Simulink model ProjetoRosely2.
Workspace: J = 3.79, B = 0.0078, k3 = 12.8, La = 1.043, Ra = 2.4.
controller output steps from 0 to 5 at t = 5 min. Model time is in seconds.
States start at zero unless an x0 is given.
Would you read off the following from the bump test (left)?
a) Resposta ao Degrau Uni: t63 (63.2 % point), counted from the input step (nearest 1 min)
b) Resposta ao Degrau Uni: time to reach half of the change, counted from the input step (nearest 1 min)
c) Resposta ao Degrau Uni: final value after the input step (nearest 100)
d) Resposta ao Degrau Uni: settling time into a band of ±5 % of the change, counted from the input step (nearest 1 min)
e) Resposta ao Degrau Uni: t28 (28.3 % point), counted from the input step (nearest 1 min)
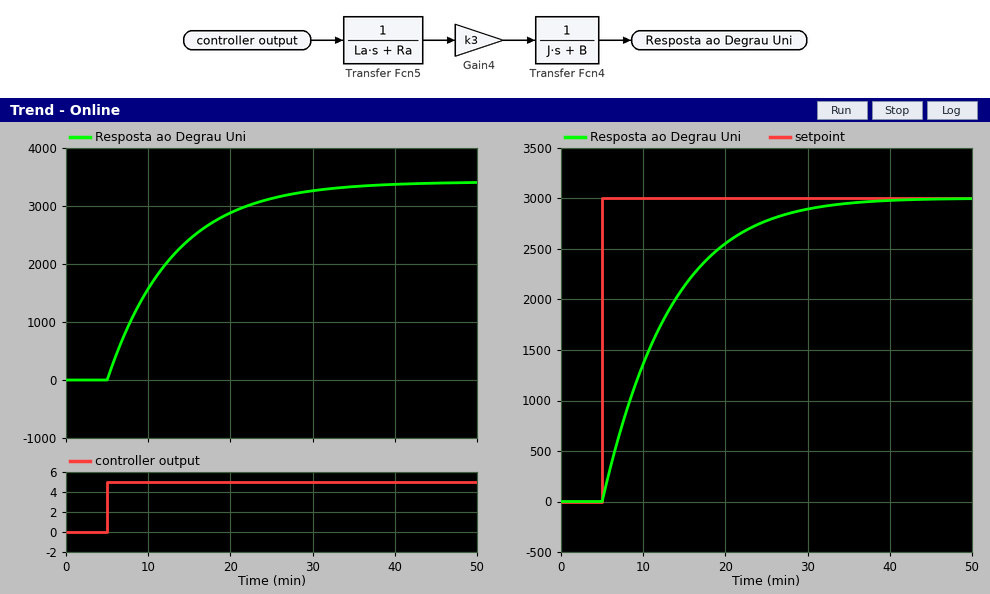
8 min
6 min
3400
24 min
3 min
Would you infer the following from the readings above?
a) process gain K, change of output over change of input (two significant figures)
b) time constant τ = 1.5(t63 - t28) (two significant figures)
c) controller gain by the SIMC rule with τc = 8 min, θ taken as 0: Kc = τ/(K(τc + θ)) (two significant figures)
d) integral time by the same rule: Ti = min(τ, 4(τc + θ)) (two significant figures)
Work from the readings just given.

680
7.5 min
0.0014
7.5 min
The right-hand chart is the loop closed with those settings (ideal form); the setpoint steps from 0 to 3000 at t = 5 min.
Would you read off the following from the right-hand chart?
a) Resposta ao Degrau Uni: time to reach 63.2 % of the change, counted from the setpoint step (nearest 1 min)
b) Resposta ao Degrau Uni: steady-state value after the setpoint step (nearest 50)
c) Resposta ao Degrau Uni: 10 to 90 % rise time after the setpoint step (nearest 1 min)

8 min
3000
17 min
